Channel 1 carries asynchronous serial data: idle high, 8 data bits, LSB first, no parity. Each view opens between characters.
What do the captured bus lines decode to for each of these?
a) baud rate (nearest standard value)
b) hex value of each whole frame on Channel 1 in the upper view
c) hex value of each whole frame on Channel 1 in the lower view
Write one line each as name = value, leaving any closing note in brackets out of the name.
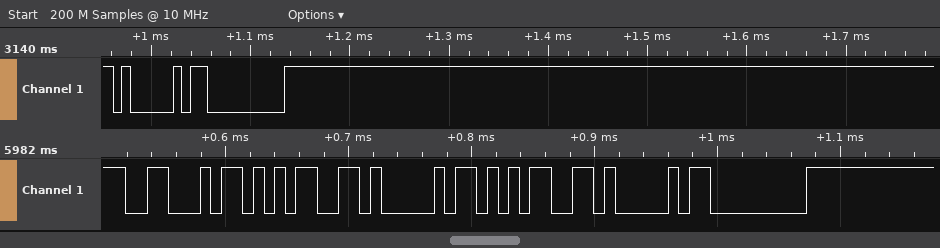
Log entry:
baud rate = 115200 baud
hex value of each whole frame on Channel 1 in the upper view = 41, 00
hex value of each whole frame on Channel 1 in the lower view = 46, 35, 41, 35, 41, 00
